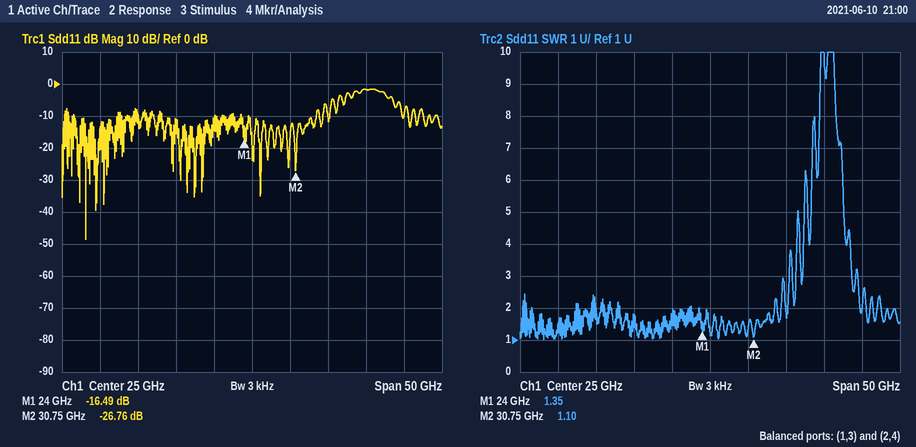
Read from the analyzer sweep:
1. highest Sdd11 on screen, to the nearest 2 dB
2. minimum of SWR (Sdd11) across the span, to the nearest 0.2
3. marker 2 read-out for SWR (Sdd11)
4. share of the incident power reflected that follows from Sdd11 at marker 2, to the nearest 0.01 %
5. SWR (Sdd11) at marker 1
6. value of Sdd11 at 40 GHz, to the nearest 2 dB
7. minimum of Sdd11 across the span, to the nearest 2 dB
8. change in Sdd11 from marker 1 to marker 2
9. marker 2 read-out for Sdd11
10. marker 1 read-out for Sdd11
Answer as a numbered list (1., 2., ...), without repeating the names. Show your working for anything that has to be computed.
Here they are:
1. -2 dB
2. 1.0
3. 1.10
4. 10^(-26.76/10) ≈ 0.21 %
5. 1.35
6. -2 dB
7. -48 dB
8. -26.76 − (-16.49) = -10.27 dB
9. -26.76 dB
10. -16.49 dB
